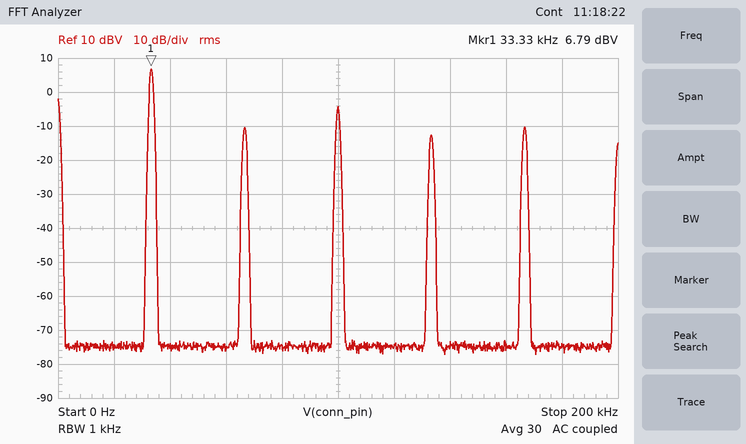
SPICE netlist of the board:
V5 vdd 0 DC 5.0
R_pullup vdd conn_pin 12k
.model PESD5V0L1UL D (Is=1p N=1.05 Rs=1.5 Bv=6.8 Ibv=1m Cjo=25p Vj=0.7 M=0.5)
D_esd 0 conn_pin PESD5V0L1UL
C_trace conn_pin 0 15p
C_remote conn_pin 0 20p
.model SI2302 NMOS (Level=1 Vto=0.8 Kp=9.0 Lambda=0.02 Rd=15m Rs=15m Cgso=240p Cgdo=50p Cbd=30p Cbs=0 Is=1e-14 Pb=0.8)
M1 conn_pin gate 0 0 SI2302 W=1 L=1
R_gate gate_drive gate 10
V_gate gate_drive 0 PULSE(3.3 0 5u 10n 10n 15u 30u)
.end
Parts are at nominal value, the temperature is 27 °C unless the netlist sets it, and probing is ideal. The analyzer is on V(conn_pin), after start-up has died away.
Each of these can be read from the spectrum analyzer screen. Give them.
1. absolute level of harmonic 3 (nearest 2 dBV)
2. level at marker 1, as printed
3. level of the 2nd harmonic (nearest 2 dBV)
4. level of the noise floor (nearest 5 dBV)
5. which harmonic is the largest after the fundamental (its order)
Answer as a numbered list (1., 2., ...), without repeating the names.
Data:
1. -4 dBV
2. 6.79 dBV
3. -10 dBV
4. -75 dBV
5. 3
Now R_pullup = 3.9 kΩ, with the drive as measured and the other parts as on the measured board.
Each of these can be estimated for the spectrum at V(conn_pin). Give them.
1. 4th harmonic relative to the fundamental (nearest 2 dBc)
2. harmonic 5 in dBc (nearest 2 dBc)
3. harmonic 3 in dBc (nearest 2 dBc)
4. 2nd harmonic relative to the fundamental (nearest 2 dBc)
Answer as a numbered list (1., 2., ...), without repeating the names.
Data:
1. -26 dBc
2. -14 dBc
3. -10 dBc
4. -26 dBc
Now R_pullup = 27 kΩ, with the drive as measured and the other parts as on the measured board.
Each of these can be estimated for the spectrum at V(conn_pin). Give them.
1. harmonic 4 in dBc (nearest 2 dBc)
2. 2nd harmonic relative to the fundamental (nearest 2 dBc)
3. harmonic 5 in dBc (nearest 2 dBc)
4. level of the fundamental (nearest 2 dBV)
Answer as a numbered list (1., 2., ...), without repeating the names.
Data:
1. -16 dBc
2. -12 dBc
3. -18 dBc
4. 6 dBV
